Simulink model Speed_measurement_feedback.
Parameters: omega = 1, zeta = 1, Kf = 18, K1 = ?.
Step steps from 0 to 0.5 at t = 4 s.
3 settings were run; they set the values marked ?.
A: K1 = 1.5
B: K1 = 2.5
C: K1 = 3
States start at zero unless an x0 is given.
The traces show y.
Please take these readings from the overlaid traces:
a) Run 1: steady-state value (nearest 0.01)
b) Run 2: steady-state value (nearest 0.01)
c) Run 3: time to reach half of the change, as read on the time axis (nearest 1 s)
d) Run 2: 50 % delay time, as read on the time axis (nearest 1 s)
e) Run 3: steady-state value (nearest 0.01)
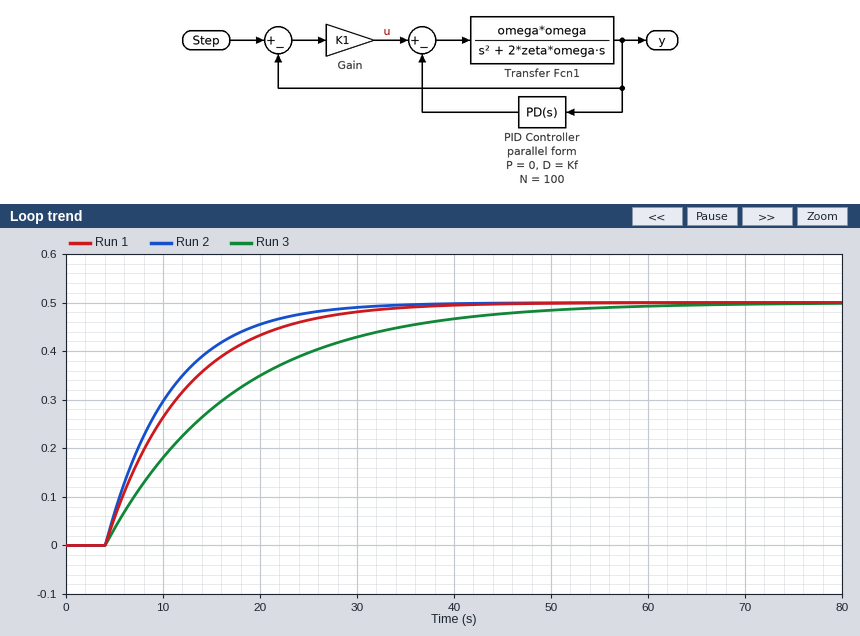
0.50
0.50
13 s
9 s
0.50
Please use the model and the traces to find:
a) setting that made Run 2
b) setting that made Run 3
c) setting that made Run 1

C
A
B
